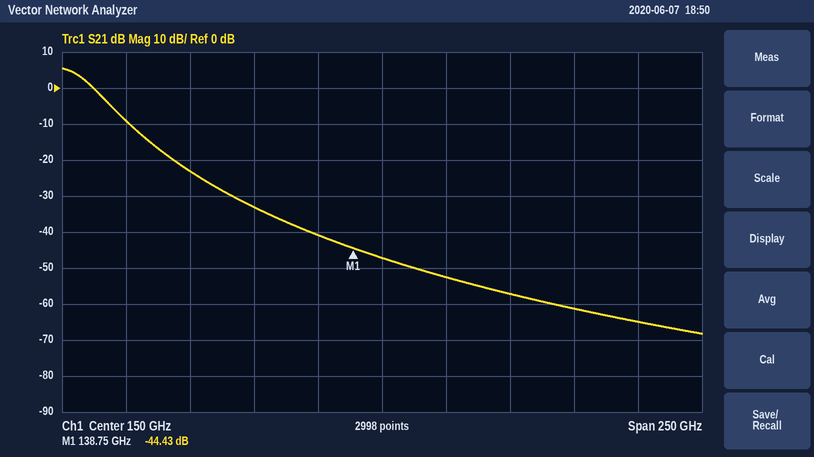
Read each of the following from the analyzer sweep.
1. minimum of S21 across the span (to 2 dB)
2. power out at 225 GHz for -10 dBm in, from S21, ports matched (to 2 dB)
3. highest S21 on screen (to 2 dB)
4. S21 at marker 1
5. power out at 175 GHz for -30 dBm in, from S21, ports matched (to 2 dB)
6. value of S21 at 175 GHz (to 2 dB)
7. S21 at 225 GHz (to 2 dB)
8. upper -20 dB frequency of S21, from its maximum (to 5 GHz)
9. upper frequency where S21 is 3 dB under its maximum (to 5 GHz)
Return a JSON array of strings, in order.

["-68 dB", "-72 dBm", "6 dB", "-44.43 dB", "-82 dBm", "-52 dB", "-62 dB", "60 GHz", "35 GHz"]
